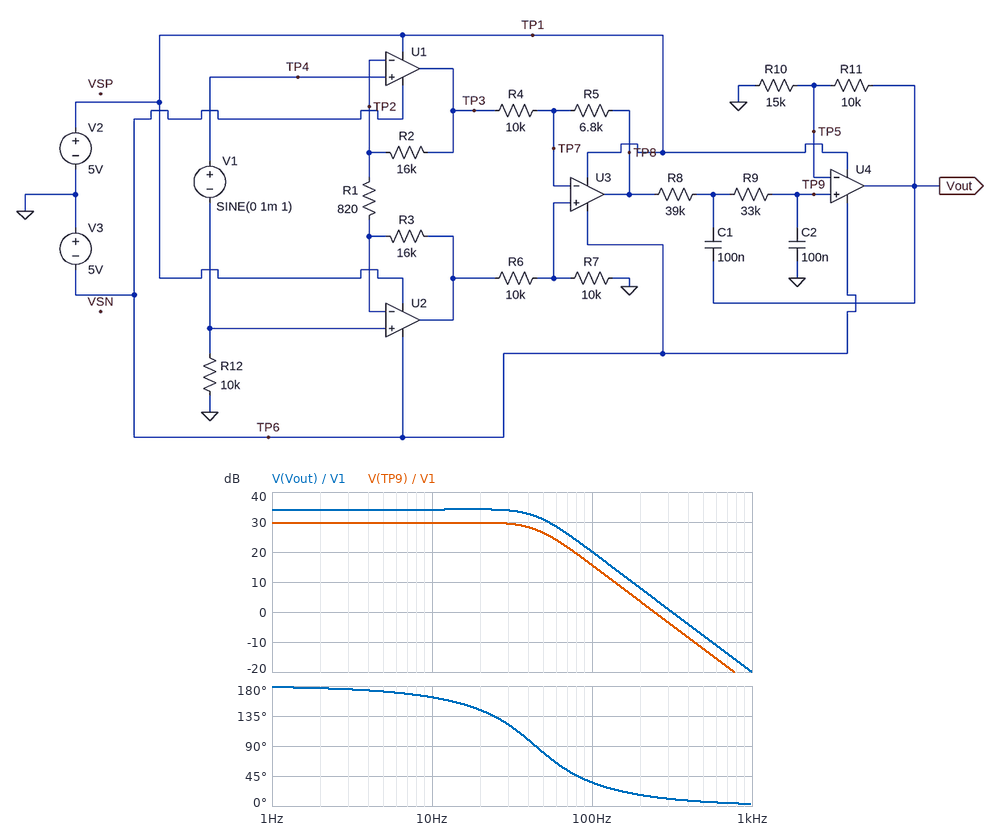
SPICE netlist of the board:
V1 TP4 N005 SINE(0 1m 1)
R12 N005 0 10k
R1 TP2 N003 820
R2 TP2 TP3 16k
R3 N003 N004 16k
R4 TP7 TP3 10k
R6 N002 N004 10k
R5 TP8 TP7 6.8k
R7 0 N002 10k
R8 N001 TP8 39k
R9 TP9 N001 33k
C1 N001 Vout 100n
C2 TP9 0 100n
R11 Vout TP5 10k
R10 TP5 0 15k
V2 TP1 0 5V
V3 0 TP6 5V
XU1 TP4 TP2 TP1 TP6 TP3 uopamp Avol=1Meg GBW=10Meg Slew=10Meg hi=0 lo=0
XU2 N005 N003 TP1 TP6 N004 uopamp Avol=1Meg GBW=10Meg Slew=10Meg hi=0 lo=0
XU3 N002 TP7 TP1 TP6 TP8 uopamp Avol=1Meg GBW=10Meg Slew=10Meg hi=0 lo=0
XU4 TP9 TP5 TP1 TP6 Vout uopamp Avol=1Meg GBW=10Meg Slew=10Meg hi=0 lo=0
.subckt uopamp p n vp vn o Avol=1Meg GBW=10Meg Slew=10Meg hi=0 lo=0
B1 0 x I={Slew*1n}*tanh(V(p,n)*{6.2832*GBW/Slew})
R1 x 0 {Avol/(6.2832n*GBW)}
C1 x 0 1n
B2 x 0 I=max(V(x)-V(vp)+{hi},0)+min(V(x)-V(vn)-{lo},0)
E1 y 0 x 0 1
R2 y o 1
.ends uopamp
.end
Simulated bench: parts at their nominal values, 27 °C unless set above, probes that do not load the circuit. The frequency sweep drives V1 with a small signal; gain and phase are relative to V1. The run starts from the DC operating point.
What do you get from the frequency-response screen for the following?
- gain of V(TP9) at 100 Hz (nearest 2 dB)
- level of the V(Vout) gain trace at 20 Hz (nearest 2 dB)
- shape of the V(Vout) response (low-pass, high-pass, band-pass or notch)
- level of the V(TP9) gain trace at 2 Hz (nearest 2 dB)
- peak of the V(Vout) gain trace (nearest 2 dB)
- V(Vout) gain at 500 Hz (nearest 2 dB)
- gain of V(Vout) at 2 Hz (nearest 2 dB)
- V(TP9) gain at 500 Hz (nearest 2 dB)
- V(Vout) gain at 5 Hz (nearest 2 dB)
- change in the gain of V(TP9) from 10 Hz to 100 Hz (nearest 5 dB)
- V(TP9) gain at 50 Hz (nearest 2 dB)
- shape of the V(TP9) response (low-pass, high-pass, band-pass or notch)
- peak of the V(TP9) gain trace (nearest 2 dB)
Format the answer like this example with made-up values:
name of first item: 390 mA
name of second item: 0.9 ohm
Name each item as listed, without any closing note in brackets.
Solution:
gain of V(TP9) at 100 Hz: 16 dB
level of the V(Vout) gain trace at 20 Hz: 34 dB
shape of the V(Vout) response: low-pass
level of the V(TP9) gain trace at 2 Hz: 30 dB
peak of the V(Vout) gain trace: 34 dB
V(Vout) gain at 500 Hz: -8 dB
gain of V(Vout) at 2 Hz: 34 dB
V(TP9) gain at 500 Hz: -12 dB
V(Vout) gain at 5 Hz: 34 dB
change in the gain of V(TP9) from 10 Hz to 100 Hz: -15 dB
V(TP9) gain at 50 Hz: 26 dB
shape of the V(TP9) response: low-pass
peak of the V(TP9) gain trace: 30 dB
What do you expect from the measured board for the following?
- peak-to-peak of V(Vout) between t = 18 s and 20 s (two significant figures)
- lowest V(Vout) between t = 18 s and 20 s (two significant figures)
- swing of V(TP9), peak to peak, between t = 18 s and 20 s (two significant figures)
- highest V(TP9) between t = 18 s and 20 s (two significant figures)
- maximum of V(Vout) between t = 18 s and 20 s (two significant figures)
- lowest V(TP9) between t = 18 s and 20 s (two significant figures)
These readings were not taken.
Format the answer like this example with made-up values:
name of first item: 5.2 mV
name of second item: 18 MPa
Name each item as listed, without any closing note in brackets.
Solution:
peak-to-peak of V(Vout) between t = 18 s and 20 s: 100 mV
lowest V(Vout) between t = 18 s and 20 s: -51 mV
swing of V(TP9), peak to peak, between t = 18 s and 20 s: 61 mV
highest V(TP9) between t = 18 s and 20 s: 30 mV
maximum of V(Vout) between t = 18 s and 20 s: 51 mV
lowest V(TP9) between t = 18 s and 20 s: -30 mV
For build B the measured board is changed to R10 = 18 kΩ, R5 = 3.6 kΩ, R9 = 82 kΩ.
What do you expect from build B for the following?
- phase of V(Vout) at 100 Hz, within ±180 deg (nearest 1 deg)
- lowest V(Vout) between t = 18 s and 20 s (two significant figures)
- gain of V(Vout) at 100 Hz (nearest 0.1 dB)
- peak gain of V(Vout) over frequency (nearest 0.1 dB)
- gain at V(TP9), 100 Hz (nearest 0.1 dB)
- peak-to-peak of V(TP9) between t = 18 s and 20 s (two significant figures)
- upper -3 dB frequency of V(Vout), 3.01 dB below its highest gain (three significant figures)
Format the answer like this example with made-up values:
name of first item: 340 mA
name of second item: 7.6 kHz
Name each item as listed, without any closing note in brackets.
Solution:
phase of V(Vout) at 100 Hz, within ±180 deg: 28 deg
lowest V(Vout) between t = 18 s and 20 s: -32 mV
gain of V(Vout) at 100 Hz: 7.7 dB
peak gain of V(Vout) over frequency: 30.1 dB
gain at V(TP9), 100 Hz: 3.9 dB
peak-to-peak of V(TP9) between t = 18 s and 20 s: 41 mV
upper -3 dB frequency of V(Vout), 3.01 dB below its highest gain: 21.7 Hz
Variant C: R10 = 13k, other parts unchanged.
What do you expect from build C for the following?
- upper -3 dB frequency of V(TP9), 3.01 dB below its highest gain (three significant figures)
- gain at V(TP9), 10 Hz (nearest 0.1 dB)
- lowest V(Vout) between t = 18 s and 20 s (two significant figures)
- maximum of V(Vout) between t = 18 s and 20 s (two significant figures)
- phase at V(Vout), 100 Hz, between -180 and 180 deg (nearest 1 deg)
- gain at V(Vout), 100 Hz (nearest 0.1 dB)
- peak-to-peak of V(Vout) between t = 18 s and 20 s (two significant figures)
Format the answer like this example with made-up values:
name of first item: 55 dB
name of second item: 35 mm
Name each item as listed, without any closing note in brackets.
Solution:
upper -3 dB frequency of V(TP9), 3.01 dB below its highest gain: 49.9 Hz
gain at V(TP9), 10 Hz: 29.8 dB
lowest V(Vout) between t = 18 s and 20 s: -54 mV
maximum of V(Vout) between t = 18 s and 20 s: 54 mV
phase at V(Vout), 100 Hz, between -180 and 180 deg: 33 deg
gain at V(Vout), 100 Hz: 20.9 dB
peak-to-peak of V(Vout) between t = 18 s and 20 s: 110 mV
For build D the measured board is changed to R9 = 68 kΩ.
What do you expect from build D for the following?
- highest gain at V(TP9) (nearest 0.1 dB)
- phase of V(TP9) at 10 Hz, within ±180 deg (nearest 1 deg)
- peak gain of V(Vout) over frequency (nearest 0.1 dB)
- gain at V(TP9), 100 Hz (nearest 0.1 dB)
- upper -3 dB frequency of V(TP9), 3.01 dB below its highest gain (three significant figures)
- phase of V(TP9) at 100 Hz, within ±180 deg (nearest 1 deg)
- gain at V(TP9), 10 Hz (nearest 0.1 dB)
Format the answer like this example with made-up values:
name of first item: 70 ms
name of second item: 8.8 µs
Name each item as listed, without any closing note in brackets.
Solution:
highest gain at V(TP9): 29.6 dB
phase of V(TP9) at 10 Hz, within ±180 deg: 150 deg
peak gain of V(Vout) over frequency: 34.1 dB
gain at V(TP9), 100 Hz: 9.0 dB
upper -3 dB frequency of V(TP9), 3.01 dB below its highest gain: 27.5 Hz
phase of V(TP9) at 100 Hz, within ±180 deg: 28 deg
gain at V(TP9), 10 Hz: 29.4 dB
